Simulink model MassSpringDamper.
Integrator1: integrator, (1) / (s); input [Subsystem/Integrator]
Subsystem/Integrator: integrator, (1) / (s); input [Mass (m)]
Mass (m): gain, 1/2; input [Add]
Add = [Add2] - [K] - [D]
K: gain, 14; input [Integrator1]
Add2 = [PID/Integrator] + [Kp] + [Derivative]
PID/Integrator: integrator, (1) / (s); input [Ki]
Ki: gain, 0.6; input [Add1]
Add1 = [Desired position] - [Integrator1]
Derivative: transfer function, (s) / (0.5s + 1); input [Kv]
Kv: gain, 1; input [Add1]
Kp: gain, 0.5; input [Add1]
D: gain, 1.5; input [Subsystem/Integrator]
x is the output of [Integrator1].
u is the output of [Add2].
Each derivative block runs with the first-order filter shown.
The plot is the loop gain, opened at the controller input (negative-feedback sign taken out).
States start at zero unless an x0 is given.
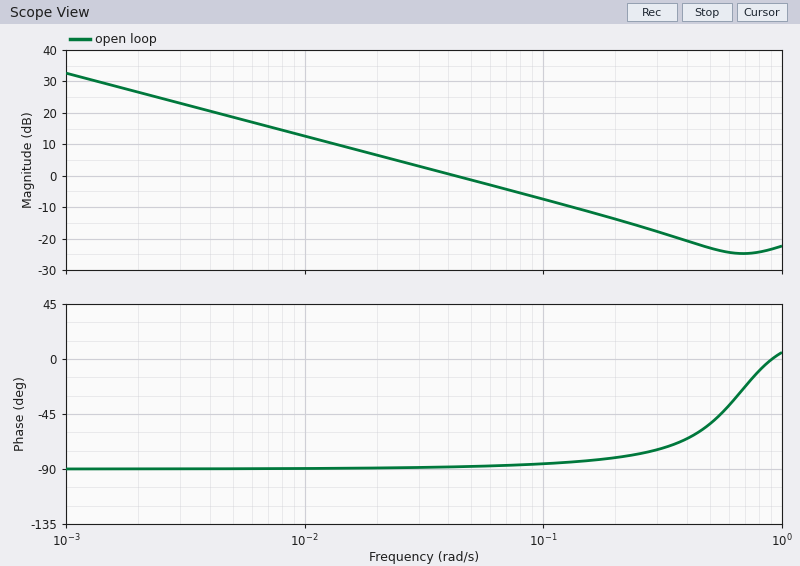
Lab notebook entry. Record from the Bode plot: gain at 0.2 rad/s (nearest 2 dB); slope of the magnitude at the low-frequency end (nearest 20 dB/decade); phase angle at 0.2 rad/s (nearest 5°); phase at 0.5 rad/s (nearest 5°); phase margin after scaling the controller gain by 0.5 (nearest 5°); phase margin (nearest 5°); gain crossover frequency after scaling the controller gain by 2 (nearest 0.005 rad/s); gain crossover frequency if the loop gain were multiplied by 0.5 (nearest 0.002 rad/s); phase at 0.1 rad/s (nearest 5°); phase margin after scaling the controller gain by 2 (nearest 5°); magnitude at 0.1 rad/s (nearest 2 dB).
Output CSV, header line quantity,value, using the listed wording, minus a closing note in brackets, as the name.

quantity,value
gain at 0.2 rad/s,-14 dB
slope of the magnitude at the low-frequency end,-20 dB/decade
phase angle at 0.2 rad/s,-80°
phase at 0.5 rad/s,-55°
phase margin after scaling the controller gain by 0.5,90°
phase margin,90°
gain crossover frequency after scaling the controller gain by 2,0.085 rad/s
gain crossover frequency if the loop gain were multiplied by 0.5,0.022 rad/s
phase at 0.1 rad/s,-85°
phase margin after scaling the controller gain by 2,95°
magnitude at 0.1 rad/s,-8 dB
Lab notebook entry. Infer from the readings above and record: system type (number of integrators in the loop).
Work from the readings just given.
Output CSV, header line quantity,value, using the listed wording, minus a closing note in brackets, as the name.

quantity,value
system type,1
